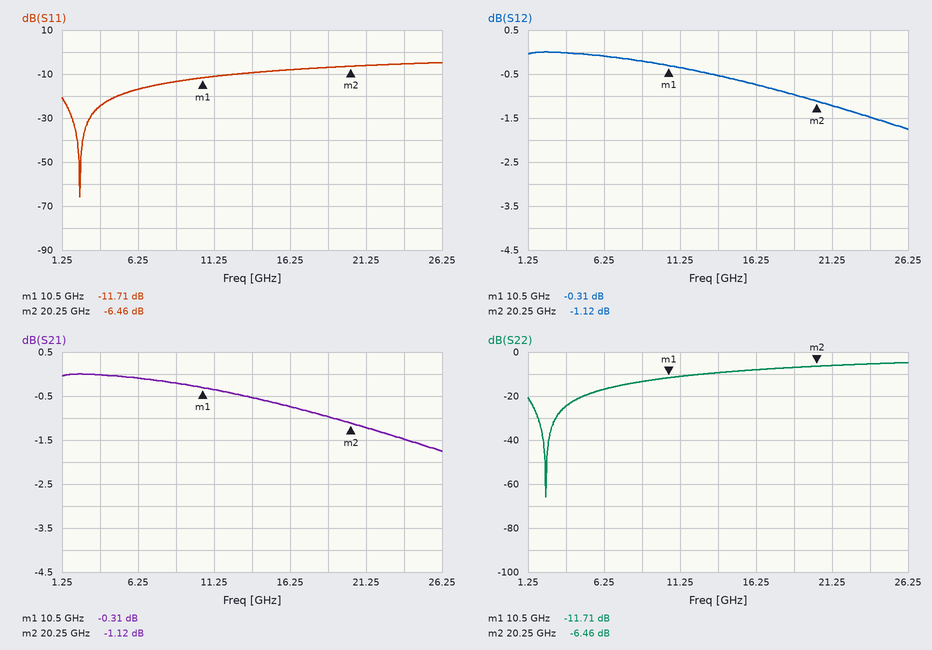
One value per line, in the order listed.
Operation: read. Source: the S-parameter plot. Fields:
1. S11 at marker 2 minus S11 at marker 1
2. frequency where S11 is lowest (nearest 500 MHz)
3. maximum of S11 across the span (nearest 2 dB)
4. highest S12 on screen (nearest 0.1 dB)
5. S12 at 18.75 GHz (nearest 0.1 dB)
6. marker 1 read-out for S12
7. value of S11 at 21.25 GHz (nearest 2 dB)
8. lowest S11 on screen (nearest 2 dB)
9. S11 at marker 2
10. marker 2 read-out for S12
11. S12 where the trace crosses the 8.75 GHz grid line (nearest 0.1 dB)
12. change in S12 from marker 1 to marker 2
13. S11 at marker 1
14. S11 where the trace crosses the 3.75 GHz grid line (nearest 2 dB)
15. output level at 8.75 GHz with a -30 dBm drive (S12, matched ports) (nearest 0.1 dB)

5.25 dB
2.5 GHz
-4 dB
0.0 dB
-1.0 dB
-0.31 dB
-6 dB
-66 dB
-6.46 dB
-1.12 dB
-0.2 dB
-0.81 dB
-11.71 dB
-24 dB
-30.2 dBm
